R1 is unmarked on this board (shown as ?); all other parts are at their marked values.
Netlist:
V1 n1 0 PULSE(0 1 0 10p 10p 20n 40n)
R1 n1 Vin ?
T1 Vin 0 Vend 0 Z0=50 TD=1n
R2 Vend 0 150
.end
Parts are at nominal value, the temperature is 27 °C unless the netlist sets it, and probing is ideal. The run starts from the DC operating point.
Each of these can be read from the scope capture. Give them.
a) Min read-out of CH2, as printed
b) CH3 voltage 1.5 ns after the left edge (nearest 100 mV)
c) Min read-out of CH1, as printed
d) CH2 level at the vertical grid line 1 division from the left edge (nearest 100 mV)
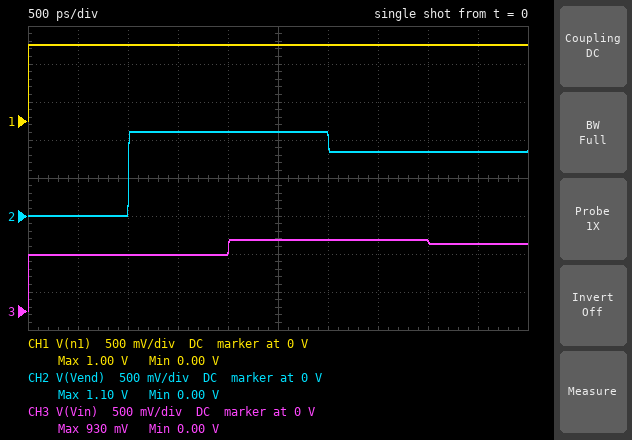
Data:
0.00 V
700 mV
0.00 V
0 V
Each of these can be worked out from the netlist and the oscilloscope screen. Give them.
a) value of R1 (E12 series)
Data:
18 Ω
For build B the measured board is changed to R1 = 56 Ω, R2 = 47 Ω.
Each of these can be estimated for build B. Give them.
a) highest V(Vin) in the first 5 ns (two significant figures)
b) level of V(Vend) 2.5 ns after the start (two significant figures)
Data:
470 mV
460 mV
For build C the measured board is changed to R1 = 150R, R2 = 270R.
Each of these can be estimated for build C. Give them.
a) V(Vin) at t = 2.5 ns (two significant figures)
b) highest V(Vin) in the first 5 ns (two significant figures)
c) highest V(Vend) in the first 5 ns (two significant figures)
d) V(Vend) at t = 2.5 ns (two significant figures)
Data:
510 mV
600 mV
570 mV
420 mV
